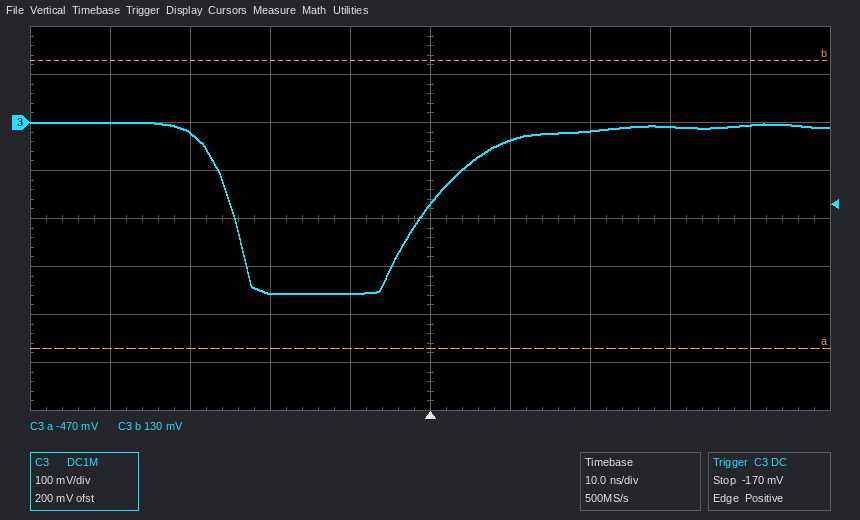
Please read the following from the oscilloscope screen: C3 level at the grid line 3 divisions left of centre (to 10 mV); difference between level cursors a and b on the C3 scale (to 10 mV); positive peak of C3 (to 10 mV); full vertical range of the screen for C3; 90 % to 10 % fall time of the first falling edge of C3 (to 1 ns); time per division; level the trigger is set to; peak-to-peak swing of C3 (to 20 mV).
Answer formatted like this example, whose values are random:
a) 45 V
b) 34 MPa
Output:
a) -20 mV
b) 600 mV
c) 0 mV
d) 800 mV
e) 6 ns
f) 10 ns
g) -170 mV
h) 360 mV
